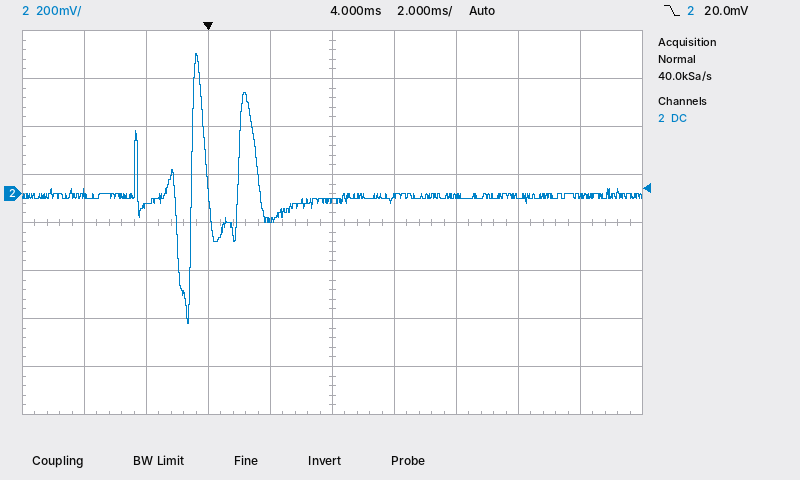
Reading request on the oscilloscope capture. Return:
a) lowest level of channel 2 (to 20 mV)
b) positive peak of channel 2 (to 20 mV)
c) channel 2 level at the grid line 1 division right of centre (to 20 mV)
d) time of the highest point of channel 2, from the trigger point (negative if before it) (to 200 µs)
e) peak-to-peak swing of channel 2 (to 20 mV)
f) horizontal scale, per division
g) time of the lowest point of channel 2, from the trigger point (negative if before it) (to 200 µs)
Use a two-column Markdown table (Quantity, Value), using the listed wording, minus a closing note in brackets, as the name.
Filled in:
| Quantity | Value |
|---|---|
| lowest level of channel 2 | -540 mV |
| positive peak of channel 2 | 580 mV |
| channel 2 level at the grid line 1 division right of centre | -20 mV |
| time of the highest point of channel 2, from the trigger point (negative if before it) | -400 µs |
| peak-to-peak swing of channel 2 | 1.12 V |
| horizontal scale, per division | 2 ms |
| time of the lowest point of channel 2, from the trigger point (negative if before it) | -600 µs |
